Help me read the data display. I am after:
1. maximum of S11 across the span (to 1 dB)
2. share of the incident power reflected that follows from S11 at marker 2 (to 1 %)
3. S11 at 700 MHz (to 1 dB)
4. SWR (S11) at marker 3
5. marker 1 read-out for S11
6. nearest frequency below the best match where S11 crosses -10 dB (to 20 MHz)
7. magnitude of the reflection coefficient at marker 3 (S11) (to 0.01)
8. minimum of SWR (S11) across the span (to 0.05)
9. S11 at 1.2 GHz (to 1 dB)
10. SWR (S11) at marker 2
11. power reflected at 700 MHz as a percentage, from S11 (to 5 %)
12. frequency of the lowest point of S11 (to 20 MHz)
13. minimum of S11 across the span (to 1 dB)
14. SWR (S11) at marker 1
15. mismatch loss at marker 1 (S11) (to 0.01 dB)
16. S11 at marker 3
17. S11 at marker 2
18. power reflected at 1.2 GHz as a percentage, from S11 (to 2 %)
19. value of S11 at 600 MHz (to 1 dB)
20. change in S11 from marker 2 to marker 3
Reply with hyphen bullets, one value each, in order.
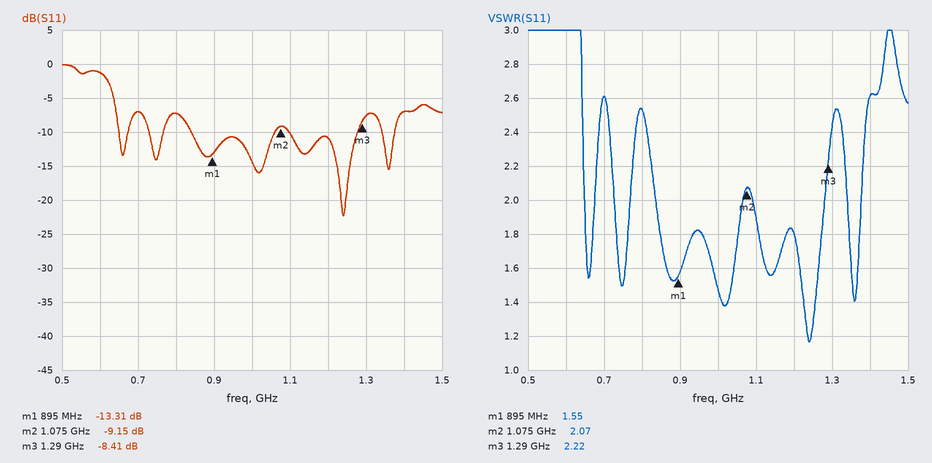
- 0 dB
- 12 %
- -7 dB
- 2.22
- -13.31 dB
- 1.10 GHz
- 0.38
- 1.15
- -11 dB
- 2.07
- 20 %
- 1.24 GHz
- -22 dB
- 1.55
- 0.21 dB
- -8.41 dB
- -9.15 dB
- 8 %
- -1 dB
- 0.74 dB
